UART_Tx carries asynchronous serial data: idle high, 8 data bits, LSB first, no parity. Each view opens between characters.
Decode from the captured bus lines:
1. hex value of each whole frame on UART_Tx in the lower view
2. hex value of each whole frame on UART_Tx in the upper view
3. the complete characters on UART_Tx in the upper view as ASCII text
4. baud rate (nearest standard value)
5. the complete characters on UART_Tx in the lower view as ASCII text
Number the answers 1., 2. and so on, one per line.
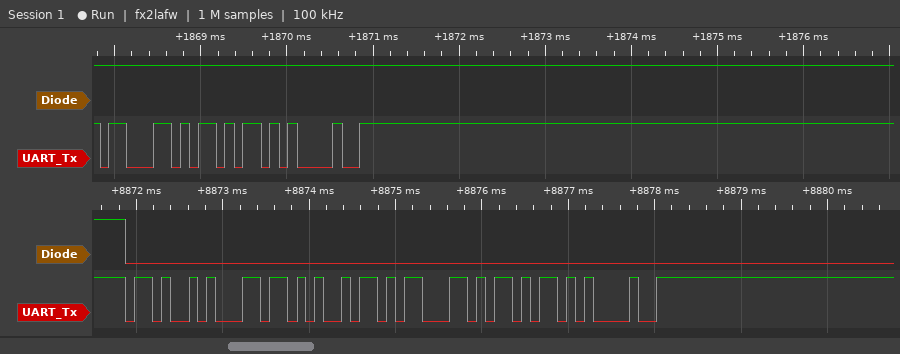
1. 4B, 6C, 69, 63, 6B, 21
2. 63, 6B, 21
3. "ck!"
4. 9600 baud
5. "Klick!"
